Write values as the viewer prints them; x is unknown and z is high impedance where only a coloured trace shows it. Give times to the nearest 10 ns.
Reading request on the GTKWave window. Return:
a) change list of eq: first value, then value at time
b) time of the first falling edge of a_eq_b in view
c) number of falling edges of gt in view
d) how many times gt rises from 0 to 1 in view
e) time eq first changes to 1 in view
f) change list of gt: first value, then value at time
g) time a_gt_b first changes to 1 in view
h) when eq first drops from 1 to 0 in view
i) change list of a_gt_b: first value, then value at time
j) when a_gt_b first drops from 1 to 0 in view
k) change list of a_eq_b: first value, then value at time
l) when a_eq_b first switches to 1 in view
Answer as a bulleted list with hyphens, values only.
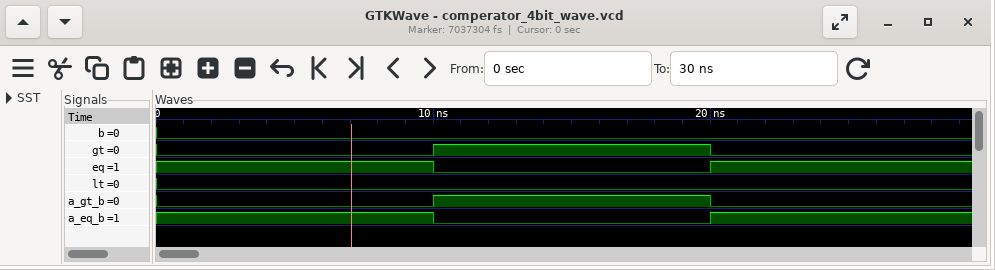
- 1, 0 at 10 ns, 1 at 20 ns
- 10 ns
- 1
- 1
- 20 ns
- 0, 1 at 10 ns, 0 at 20 ns
- 10 ns
- 10 ns
- 0, 1 at 10 ns, 0 at 20 ns
- 20 ns
- 1, 0 at 10 ns, 1 at 20 ns
- 20 ns
